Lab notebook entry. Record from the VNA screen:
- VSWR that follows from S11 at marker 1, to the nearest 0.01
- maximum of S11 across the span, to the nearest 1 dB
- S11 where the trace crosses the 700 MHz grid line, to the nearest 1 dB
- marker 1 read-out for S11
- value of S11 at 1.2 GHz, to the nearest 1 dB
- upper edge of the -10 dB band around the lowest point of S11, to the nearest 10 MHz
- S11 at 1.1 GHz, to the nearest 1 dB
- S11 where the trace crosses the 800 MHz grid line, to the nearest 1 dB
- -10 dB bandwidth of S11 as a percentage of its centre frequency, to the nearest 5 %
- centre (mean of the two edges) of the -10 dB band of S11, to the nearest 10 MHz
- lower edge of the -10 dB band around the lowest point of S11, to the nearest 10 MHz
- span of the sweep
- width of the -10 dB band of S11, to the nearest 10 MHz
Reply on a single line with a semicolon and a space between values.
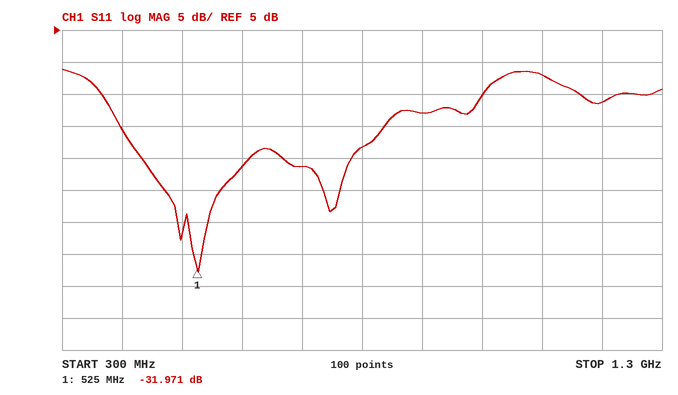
1.05; -1 dB; -16 dB; -31.971 dB; -6 dB; 840 MHz; -2 dB; -13 dB; 70 %; 620 MHz; 400 MHz; 1 GHz; 440 MHz
